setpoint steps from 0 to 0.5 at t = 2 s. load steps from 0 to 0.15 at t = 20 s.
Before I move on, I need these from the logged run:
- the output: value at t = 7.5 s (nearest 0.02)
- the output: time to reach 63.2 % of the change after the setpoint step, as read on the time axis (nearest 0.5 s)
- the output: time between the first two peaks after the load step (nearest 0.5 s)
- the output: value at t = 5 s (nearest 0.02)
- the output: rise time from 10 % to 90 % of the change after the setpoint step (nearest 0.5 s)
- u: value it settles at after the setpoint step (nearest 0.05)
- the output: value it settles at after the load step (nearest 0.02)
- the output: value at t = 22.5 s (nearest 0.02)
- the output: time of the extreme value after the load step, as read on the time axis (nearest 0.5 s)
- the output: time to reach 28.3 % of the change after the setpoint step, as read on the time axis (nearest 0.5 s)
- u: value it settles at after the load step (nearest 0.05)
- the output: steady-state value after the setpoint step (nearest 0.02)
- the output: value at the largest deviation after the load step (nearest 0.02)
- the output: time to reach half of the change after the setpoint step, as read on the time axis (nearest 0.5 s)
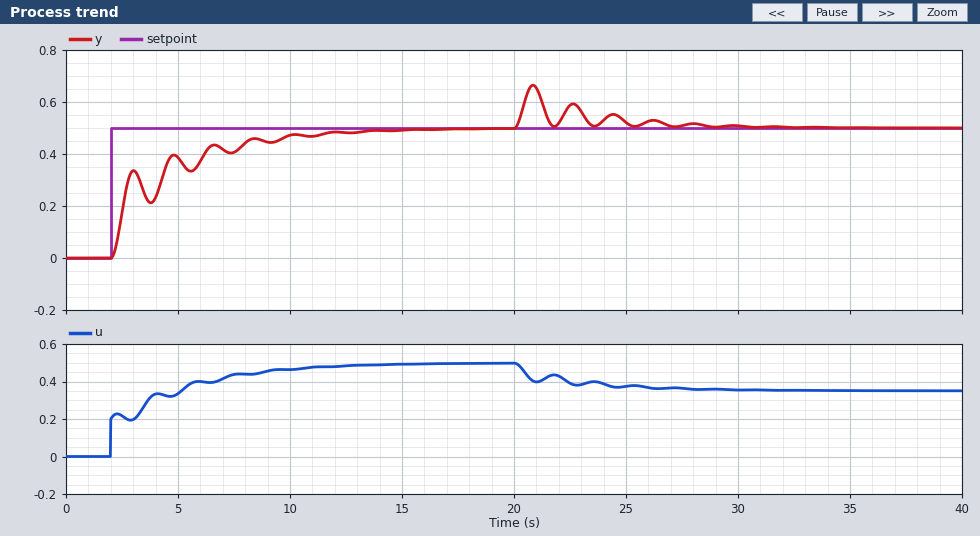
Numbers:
0.40
3.0 s
2.0 s
0.38
6.0 s
0.50
0.50
0.58
21.0 s
2.5 s
0.35
0.50
0.66
2.5 s
